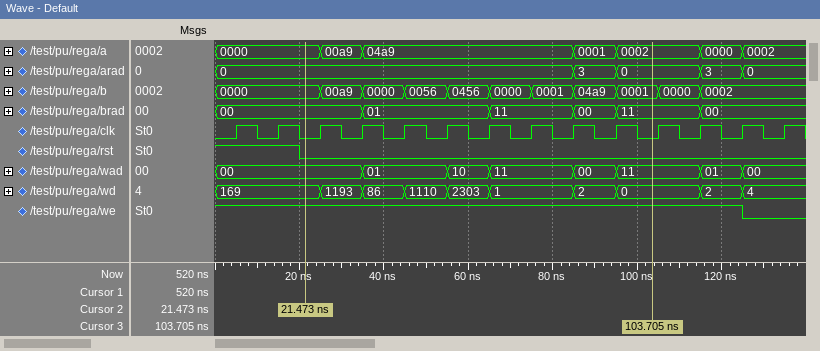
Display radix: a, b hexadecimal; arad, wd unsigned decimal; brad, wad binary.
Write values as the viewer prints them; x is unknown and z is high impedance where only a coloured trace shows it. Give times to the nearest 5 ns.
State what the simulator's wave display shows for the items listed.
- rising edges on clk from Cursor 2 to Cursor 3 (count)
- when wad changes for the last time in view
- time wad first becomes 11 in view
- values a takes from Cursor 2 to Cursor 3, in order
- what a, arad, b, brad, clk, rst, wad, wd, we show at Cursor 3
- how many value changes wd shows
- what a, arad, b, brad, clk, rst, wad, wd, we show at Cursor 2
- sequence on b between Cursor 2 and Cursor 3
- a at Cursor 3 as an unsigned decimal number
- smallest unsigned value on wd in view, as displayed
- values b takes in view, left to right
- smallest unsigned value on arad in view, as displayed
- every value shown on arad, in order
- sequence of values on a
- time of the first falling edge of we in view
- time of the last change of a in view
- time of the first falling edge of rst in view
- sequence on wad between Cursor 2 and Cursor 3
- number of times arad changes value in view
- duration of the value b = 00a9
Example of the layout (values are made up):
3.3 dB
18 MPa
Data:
8
125 ns
65 ns
0000, 00a9, 04a9, 0001, 0002
a=0002, arad=0, b=0001, brad=11, clk=0, rst=0, wad=11, wd=0, we=1
9
a=0000, arad=0, b=0000, brad=00, clk=0, rst=0, wad=00, wd=169, we=1
0000, 00a9, 0000, 0056, 0456, 0000, 0001, 04a9, 0001
2
0
0000, 00a9, 0000, 0056, 0456, 0000, 0001, 04a9, 0001, 0000, 0002
0
0, 3, 0, 3, 0
0000, 00a9, 04a9, 0001, 0002, 0000, 0002
125 ns
125 ns
20 ns
00, 01, 10, 11, 00, 11
4
10 ns
